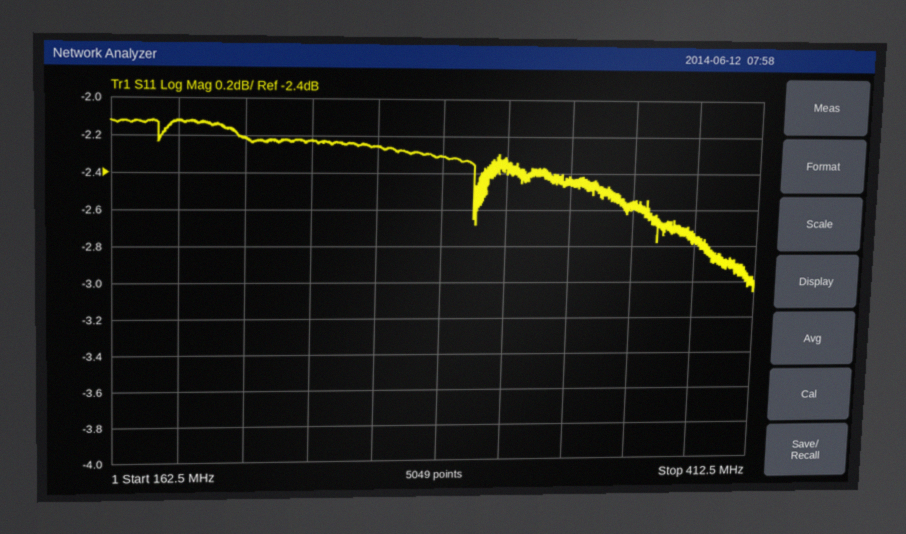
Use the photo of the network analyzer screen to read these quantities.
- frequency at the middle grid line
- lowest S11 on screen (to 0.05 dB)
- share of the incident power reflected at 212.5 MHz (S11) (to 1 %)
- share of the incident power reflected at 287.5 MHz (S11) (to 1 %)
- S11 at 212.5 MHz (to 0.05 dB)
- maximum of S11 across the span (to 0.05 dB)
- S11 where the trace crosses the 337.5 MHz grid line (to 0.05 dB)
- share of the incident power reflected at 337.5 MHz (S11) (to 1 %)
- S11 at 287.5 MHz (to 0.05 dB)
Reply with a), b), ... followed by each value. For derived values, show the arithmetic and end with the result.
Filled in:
a) 287.5 MHz
b) -3.05 dB
c) 10^(-2.2/10) ≈ 60 %
d) 10^(-2.3/10) ≈ 59 %
e) -2.20 dB
f) -2.10 dB
g) -2.45 dB
h) 10^(-2.45/10) ≈ 57 %
i) -2.30 dB
